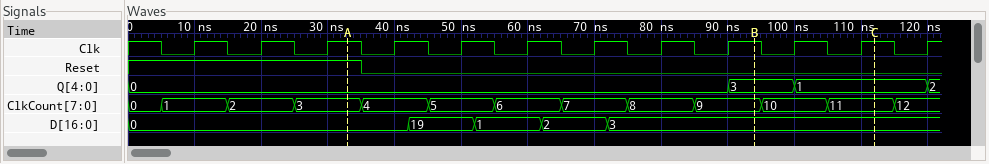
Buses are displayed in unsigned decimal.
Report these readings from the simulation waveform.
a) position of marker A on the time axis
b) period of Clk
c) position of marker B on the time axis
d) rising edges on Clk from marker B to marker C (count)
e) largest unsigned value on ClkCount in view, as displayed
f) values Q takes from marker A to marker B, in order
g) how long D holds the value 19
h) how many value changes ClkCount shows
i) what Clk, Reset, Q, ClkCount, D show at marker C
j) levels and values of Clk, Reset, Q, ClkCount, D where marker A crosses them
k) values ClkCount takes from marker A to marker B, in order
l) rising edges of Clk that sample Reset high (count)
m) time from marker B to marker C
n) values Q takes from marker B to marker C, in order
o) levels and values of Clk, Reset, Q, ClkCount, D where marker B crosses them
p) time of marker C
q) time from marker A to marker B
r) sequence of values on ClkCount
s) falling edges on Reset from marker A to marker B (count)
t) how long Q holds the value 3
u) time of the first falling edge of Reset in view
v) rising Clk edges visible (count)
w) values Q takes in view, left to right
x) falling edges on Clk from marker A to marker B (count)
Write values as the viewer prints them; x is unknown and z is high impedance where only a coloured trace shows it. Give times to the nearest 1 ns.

33 ns
10 ns
94 ns
2
12
0, 3
10 ns
12
Clk=1, Reset=0, Q=1, ClkCount=11, D=3
Clk=1, Reset=1, Q=0, ClkCount=3, D=0
3, 4, 5, 6, 7, 8, 9
3
18 ns
3, 1
Clk=1, Reset=0, Q=3, ClkCount=9, D=3
112 ns
61 ns
0, 1, 2, 3, 4, 5, 6, 7, 8, 9, 10, 11, 12
1
10 ns
35 ns
12
0, 3, 1, 2
6
